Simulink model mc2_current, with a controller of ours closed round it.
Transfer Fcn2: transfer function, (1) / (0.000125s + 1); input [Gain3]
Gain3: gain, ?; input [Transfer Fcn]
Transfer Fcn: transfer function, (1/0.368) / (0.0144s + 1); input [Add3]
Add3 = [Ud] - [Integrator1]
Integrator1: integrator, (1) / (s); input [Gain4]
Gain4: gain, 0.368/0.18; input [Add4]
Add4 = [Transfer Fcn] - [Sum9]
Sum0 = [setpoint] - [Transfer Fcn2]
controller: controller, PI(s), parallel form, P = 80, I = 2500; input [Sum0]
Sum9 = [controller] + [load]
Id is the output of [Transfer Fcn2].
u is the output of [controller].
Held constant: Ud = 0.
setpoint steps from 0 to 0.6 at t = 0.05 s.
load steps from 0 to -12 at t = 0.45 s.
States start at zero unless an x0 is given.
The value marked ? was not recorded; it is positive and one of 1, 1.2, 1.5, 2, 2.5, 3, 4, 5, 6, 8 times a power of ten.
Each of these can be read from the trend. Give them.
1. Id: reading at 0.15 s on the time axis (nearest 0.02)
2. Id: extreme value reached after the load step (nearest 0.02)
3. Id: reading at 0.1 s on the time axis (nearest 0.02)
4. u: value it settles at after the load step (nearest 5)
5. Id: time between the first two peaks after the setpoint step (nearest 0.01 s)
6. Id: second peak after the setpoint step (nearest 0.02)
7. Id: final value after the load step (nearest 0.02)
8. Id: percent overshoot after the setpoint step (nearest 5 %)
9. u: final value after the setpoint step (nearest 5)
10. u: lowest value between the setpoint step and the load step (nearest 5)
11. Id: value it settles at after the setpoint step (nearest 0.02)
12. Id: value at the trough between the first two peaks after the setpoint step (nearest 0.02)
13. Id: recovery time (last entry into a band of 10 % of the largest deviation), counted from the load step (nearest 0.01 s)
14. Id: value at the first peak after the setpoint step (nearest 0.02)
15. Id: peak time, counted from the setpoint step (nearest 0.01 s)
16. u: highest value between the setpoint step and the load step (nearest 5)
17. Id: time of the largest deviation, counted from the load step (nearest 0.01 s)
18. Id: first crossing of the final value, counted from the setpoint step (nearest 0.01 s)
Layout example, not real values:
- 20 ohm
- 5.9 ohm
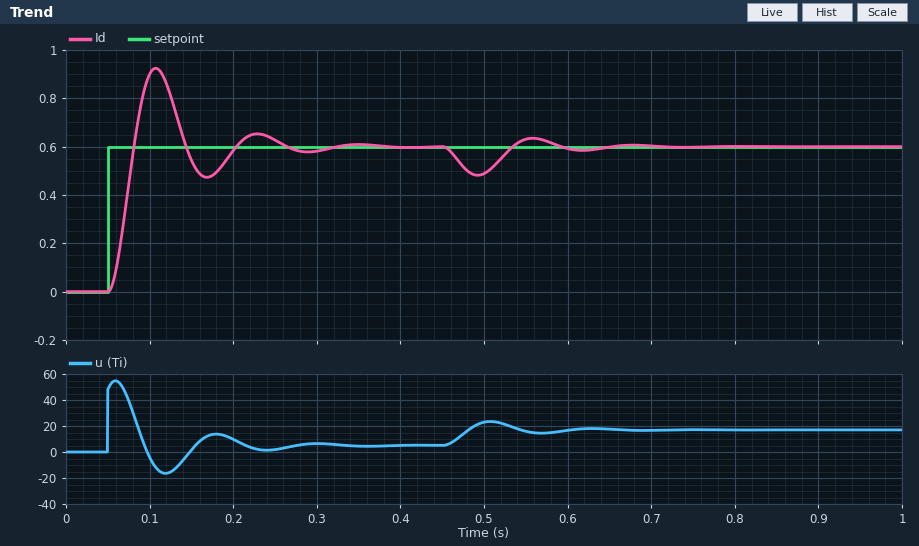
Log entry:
- 0.54
- 0.48
- 0.90
- 15
- 0.12 s
- 0.66
- 0.60
- 55 %
- 5
- -15
- 0.60
- 0.48
- 0.18 s
- 0.92
- 0.06 s
- 55
- 0.04 s
- 0.03 s
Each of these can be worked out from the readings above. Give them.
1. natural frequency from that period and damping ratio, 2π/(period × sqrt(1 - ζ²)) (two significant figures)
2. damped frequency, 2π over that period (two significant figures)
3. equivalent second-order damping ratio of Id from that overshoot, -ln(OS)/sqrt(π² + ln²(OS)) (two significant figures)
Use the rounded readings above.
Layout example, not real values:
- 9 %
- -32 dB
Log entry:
- 53 rad/s
- 52 rad/s
- 0.19
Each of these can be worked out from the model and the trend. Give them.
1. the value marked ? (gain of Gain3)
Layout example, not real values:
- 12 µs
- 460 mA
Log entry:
- 0.12
